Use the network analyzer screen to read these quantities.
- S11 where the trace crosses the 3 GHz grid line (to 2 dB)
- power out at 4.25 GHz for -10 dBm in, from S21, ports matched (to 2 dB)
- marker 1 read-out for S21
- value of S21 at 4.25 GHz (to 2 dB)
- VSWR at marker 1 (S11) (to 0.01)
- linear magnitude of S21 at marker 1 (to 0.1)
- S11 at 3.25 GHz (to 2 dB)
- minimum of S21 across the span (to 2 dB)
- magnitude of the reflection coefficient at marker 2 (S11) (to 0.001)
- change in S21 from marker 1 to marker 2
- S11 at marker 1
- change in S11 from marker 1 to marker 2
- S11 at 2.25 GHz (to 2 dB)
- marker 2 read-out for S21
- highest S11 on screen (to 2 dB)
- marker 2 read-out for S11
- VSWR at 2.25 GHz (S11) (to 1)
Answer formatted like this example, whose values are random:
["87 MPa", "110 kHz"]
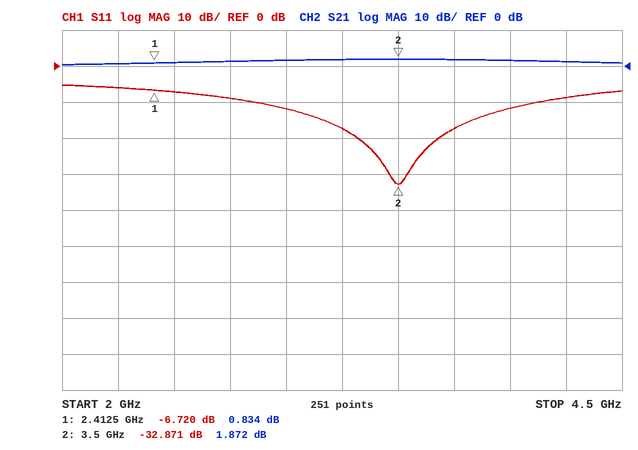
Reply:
["-12 dB", "-8 dBm", "0.834 dB", "2 dB", "2.71", "1.1", "-18 dB", "0 dB", "0.023", "1.038 dB", "-6.720 dB", "-26.151 dB", "-6 dB", "1.872 dB", "-6 dB", "-32.871 dB", "3"]
